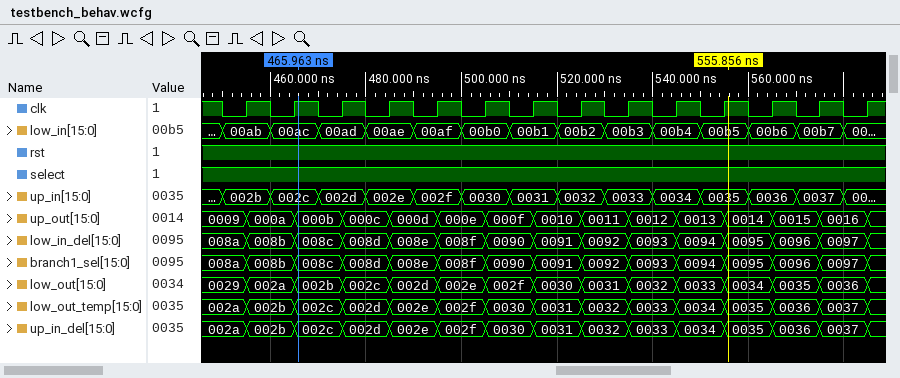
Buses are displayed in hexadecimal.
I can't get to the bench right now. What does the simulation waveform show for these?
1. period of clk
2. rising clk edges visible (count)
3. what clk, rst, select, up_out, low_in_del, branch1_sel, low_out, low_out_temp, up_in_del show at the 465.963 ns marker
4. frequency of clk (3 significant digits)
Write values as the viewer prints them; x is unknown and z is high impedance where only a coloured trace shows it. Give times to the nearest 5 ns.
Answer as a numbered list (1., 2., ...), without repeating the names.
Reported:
1. 10 ns
2. 14
3. clk=1, rst=1, select=1, up_out=000b, low_in_del=008c, branch1_sel=008c, low_out=002b, low_out_temp=002c, up_in_del=002c
4. 100 MHz
